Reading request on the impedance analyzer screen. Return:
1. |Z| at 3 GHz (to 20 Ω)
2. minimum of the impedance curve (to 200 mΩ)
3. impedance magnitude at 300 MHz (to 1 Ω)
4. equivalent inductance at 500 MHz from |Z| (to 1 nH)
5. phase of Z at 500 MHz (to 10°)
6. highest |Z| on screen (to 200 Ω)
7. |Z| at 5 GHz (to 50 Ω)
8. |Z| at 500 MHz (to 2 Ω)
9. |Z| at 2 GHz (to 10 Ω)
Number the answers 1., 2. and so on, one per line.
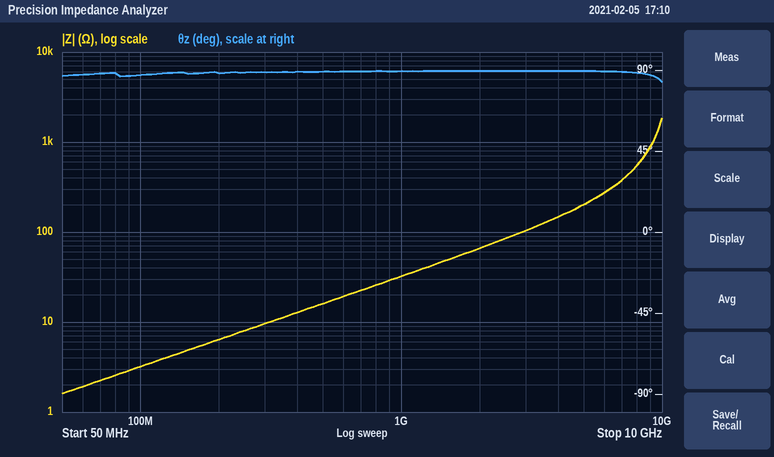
1. 100 Ω
2. 1.6 Ω
3. 10 Ω
4. 5 nH
5. 90°
6. 1.8 kΩ
7. 200 Ω
8. 16 Ω
9. 70 Ω
